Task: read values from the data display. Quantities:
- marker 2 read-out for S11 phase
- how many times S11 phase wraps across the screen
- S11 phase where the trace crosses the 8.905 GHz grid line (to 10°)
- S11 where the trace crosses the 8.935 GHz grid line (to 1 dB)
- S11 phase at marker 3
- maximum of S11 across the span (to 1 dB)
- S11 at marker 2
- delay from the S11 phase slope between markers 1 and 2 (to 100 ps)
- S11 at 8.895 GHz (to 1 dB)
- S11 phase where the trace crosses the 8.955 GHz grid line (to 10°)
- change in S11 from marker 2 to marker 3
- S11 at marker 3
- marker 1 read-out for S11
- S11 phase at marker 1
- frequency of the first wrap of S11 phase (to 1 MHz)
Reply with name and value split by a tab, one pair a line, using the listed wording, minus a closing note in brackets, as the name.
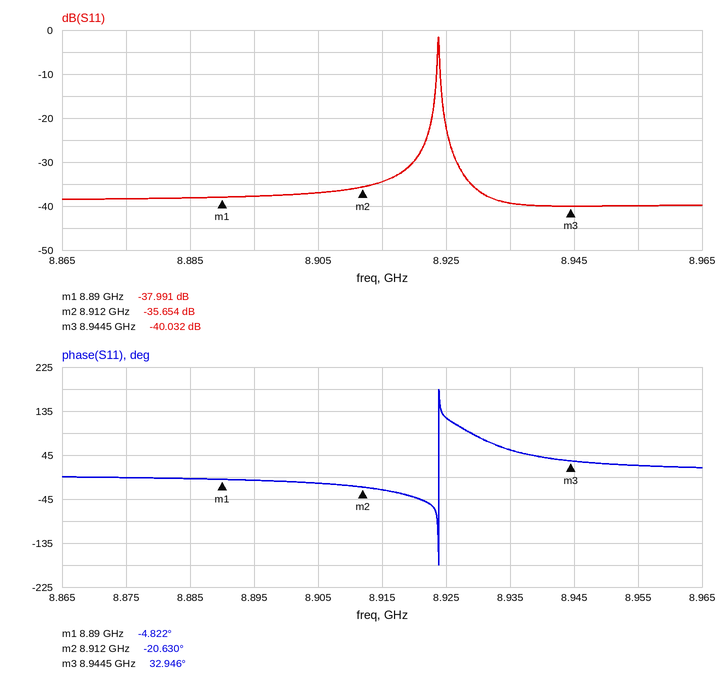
marker 2 read-out for S11 phase	-20.630°
how many times S11 phase wraps across the screen	1
S11 phase where the trace crosses the 8.905 GHz grid line	-10°
S11 where the trace crosses the 8.935 GHz grid line	-39 dB
S11 phase at marker 3	32.946°
maximum of S11 across the span	-2 dB
S11 at marker 2	-35.654 dB
delay from the S11 phase slope between markers 1 and 2	2.0 ns
S11 at 8.895 GHz	-38 dB
S11 phase where the trace crosses the 8.955 GHz grid line	20°
change in S11 from marker 2 to marker 3	-4.378 dB
S11 at marker 3	-40.032 dB
marker 1 read-out for S11	-37.991 dB
S11 phase at marker 1	-4.822°
frequency of the first wrap of S11 phase	8.924 GHz
